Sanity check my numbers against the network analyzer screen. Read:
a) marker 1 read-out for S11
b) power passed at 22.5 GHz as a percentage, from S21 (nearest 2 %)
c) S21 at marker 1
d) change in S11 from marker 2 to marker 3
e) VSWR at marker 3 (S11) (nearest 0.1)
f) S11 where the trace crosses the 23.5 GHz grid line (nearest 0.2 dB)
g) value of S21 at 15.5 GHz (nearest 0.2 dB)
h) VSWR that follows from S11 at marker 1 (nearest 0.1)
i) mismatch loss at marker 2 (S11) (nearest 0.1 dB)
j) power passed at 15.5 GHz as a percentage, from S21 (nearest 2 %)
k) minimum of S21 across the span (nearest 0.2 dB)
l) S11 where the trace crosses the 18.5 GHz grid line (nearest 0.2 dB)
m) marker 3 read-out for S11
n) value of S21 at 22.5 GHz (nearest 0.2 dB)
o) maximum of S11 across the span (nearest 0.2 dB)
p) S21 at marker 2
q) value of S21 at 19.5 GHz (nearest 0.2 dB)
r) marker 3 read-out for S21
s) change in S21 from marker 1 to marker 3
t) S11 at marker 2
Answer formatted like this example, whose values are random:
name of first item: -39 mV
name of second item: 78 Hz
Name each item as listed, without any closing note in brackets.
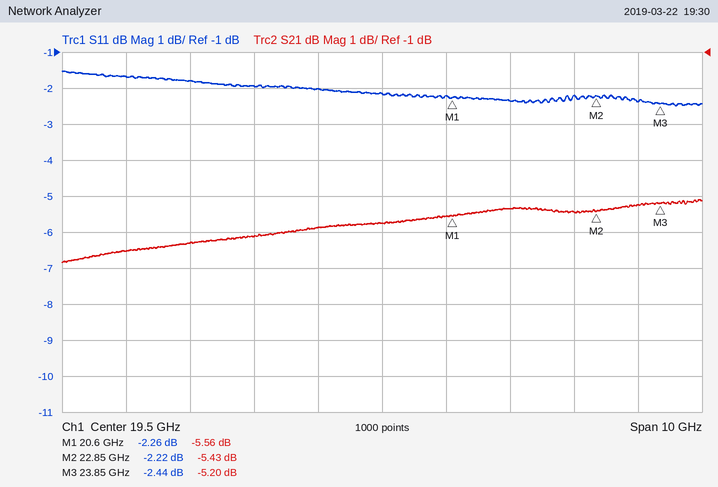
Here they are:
marker 1 read-out for S11: -2.26 dB
power passed at 22.5 GHz as a percentage, from S21: 28 %
S21 at marker 1: -5.56 dB
change in S11 from marker 2 to marker 3: -0.22 dB
VSWR at marker 3 (S11): 7.2
S11 where the trace crosses the 23.5 GHz grid line: -2.4 dB
value of S21 at 15.5 GHz: -6.6 dB
VSWR that follows from S11 at marker 1: 7.7
mismatch loss at marker 2 (S11): 4.0 dB
power passed at 15.5 GHz as a percentage, from S21: 22 %
minimum of S21 across the span: -6.8 dB
S11 where the trace crosses the 18.5 GHz grid line: -2.0 dB
marker 3 read-out for S11: -2.44 dB
value of S21 at 22.5 GHz: -5.4 dB
maximum of S11 across the span: -1.6 dB
S21 at marker 2: -5.43 dB
value of S21 at 19.5 GHz: -5.8 dB
marker 3 read-out for S21: -5.20 dB
change in S21 from marker 1 to marker 3: 0.36 dB
S11 at marker 2: -2.22 dB
